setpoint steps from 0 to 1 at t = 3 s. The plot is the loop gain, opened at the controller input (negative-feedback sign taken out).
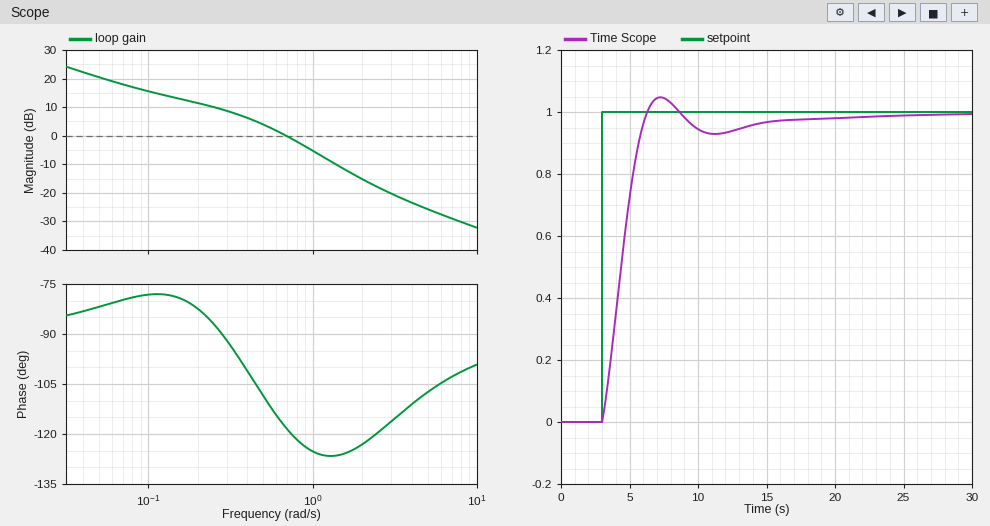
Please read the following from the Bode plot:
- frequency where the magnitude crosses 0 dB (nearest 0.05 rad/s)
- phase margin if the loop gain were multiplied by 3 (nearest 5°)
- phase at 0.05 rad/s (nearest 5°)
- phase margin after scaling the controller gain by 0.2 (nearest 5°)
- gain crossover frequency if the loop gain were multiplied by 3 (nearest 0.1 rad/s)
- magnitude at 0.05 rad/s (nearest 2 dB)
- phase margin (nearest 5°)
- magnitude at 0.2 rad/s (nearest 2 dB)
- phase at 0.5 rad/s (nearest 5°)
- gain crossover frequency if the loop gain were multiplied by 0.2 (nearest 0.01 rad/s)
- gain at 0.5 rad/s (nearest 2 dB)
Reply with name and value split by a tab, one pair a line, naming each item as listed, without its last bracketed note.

frequency where the magnitude crosses 0 dB	0.70 rad/s
phase margin if the loop gain were multiplied by 3	55°
phase at 0.05 rad/s	-80°
phase margin after scaling the controller gain by 0.2	100°
gain crossover frequency if the loop gain were multiplied by 3	1.3 rad/s
magnitude at 0.05 rad/s	20 dB
phase margin	60°
magnitude at 0.2 rad/s	12 dB
phase at 0.5 rad/s	-110°
gain crossover frequency if the loop gain were multiplied by 0.2	0.13 rad/s
gain at 0.5 rad/s	4 dB
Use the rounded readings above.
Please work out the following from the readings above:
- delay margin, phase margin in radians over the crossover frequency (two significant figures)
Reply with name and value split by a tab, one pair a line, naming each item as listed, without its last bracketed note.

delay margin, phase margin in radians over the crossover frequency	1.5 s
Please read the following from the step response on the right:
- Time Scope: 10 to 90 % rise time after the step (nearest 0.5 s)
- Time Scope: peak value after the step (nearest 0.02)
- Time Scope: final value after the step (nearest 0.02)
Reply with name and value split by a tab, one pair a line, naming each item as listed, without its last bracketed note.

Time Scope: 10 to 90 % rise time after the step	2.5 s
Time Scope: peak value after the step	1.04
Time Scope: final value after the step	1.00
